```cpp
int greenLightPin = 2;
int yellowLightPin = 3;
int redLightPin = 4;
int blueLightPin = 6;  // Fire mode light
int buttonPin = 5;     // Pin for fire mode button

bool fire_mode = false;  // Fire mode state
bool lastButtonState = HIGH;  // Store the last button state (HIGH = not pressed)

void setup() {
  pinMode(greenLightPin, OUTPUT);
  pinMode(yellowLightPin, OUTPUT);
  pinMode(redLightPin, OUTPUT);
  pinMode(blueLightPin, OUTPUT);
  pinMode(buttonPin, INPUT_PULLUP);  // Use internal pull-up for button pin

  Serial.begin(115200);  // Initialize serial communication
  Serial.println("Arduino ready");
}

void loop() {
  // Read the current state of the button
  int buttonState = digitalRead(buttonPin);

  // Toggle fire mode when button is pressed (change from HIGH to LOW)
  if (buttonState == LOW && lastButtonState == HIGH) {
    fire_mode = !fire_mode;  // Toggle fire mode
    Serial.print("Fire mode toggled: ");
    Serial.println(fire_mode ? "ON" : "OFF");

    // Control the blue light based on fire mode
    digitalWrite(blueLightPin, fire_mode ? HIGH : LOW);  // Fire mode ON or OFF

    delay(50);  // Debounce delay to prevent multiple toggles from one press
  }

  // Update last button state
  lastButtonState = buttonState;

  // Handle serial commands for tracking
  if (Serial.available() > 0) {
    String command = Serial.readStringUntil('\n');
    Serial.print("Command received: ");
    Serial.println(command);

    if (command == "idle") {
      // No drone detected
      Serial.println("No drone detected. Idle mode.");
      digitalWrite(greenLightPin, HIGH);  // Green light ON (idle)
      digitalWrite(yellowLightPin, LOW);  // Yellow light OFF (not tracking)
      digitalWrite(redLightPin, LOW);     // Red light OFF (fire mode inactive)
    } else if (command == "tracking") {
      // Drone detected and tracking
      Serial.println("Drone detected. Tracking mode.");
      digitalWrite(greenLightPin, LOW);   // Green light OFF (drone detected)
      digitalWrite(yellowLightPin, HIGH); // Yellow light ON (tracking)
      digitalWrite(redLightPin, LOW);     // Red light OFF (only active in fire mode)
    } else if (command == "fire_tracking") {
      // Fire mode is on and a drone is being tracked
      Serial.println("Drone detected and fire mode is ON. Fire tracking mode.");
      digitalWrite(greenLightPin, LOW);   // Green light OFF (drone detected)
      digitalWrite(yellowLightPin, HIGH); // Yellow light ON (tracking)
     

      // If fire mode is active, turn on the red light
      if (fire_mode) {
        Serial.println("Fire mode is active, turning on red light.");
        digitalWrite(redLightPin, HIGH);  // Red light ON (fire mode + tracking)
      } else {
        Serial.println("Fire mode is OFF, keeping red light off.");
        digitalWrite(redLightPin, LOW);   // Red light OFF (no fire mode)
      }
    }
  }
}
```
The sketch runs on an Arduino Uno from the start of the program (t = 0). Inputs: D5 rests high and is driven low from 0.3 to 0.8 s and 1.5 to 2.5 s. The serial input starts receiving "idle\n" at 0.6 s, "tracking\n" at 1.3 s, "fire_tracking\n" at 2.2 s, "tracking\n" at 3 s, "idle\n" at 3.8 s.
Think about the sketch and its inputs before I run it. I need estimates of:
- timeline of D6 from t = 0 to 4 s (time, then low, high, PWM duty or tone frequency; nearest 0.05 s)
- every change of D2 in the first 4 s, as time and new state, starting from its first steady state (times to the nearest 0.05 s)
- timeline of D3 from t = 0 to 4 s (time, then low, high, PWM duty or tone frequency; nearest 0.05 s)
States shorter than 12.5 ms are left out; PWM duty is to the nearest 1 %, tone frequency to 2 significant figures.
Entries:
0 s low; 0.3 s high; 1.5 s low
0 s low; 0.6 s high; 1.3 s low; 3.8 s high
0 s low; 1.3 s high; 3.8 s low
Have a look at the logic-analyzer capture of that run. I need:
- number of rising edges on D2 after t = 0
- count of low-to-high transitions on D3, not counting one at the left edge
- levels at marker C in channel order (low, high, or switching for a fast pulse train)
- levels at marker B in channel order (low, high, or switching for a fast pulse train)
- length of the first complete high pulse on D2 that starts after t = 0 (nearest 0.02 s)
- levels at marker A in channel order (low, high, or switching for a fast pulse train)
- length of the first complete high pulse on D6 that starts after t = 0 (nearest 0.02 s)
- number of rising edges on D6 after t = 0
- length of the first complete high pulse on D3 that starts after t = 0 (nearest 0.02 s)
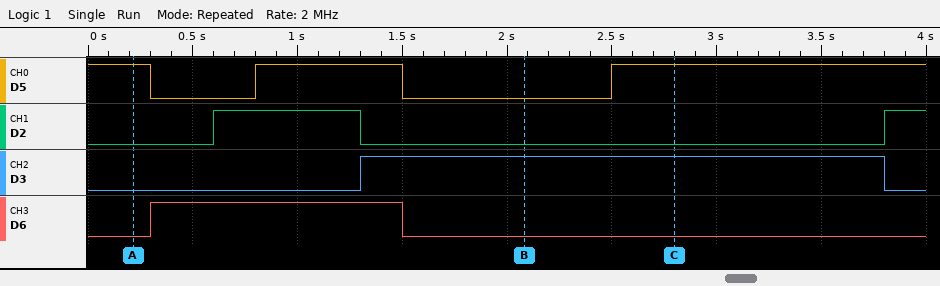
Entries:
2
1
D5 high, D2 low, D3 high, D6 low
D5 low, D2 low, D3 high, D6 low
0.70 s
D5 high, D2 low, D3 low, D6 low
1.20 s
1
2.50 s
